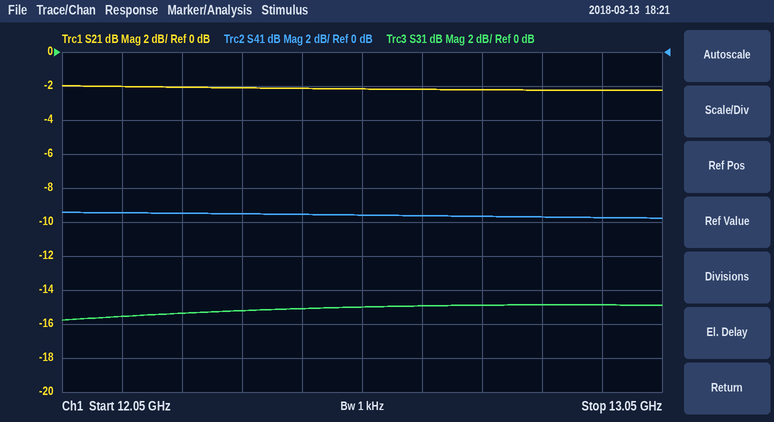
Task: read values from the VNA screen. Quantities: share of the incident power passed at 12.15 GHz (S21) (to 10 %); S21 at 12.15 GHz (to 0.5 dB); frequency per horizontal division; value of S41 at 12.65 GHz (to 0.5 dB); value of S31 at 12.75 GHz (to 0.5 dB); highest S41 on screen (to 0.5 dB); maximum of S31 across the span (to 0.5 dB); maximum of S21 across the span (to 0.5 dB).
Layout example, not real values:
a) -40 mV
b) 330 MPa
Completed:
a) 60 %
b) -2.0 dB
c) 100 MHz
d) -9.5 dB
e) -15.0 dB
f) -9.5 dB
g) -15.0 dB
h) -2.0 dB
